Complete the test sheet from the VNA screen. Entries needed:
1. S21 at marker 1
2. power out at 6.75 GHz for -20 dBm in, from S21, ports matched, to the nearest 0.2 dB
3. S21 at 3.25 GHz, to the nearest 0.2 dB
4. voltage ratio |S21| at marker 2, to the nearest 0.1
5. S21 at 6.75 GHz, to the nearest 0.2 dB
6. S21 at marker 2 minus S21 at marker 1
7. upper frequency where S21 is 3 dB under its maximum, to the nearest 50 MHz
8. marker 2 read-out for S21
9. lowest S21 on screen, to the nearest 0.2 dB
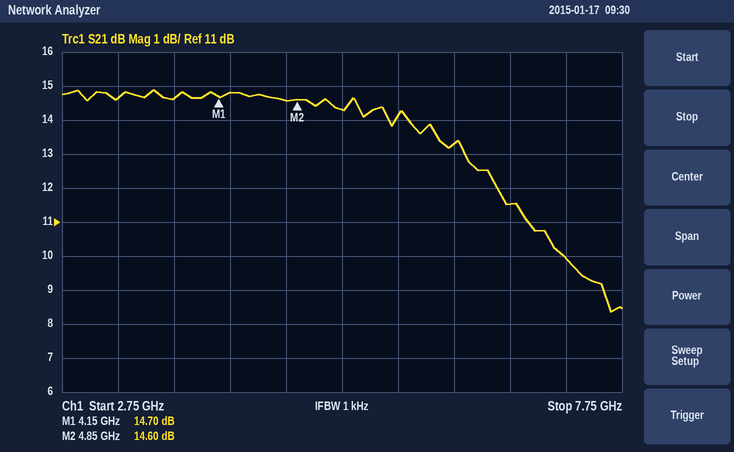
14.70 dB
-8.4 dBm
14.6 dB
5.4
11.6 dB
-0.10 dB
6.65 GHz
14.60 dB
8.4 dB
